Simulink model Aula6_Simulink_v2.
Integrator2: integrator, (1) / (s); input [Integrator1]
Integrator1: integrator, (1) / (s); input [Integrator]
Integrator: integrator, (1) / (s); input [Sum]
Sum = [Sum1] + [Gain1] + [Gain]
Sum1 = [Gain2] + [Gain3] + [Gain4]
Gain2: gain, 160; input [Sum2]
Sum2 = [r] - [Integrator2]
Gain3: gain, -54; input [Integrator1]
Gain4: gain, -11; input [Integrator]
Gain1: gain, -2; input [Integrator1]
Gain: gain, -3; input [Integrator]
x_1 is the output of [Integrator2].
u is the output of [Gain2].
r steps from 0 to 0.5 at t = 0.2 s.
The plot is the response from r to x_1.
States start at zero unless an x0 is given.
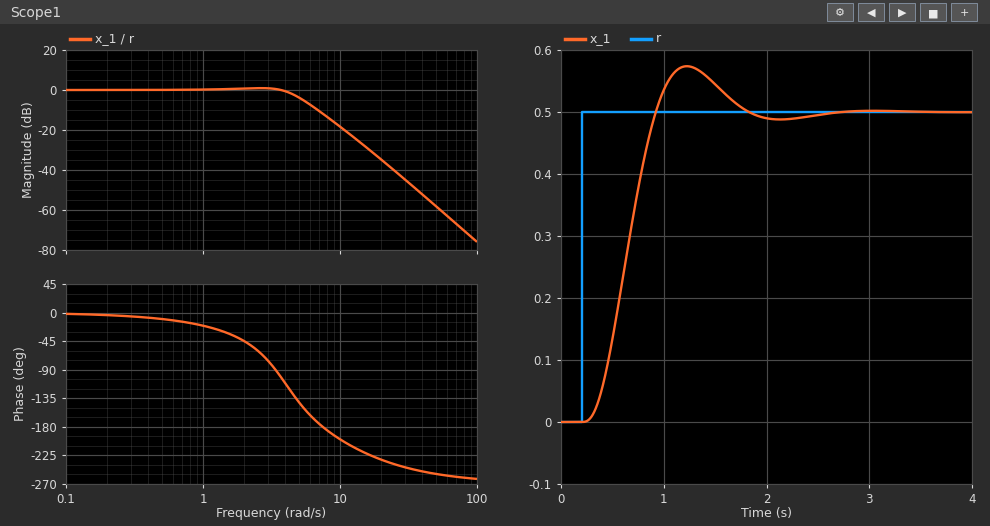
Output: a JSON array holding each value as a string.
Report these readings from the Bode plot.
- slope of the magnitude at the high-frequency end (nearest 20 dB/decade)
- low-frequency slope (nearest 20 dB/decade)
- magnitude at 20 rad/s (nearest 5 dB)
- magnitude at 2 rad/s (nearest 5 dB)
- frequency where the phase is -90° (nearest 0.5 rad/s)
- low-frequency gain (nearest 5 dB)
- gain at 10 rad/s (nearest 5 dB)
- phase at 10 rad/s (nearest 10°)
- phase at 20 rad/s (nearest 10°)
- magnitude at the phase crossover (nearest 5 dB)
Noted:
["-60 dB/decade", "0 dB/decade", "-35 dB", "0 dB", "3.5 rad/s", "0 dB", "-20 dB", "-200°", "-230°", "-10 dB"]
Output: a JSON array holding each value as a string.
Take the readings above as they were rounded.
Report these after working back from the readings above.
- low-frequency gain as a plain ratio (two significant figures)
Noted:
["1.0"]
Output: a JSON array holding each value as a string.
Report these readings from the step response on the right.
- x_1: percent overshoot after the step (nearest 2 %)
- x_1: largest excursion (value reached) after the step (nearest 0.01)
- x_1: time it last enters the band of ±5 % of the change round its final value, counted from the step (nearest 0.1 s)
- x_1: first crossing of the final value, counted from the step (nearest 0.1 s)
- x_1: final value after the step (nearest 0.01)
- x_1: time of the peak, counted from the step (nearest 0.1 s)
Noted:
["14 %", "0.57", "1.4 s", "0.7 s", "0.50", "1.0 s"]
